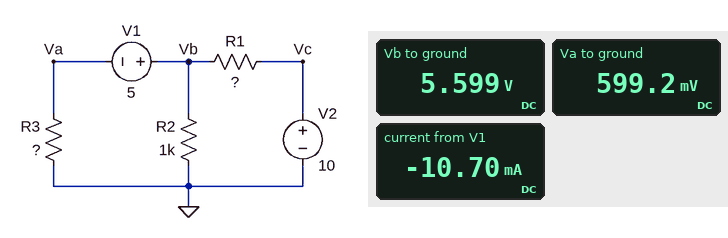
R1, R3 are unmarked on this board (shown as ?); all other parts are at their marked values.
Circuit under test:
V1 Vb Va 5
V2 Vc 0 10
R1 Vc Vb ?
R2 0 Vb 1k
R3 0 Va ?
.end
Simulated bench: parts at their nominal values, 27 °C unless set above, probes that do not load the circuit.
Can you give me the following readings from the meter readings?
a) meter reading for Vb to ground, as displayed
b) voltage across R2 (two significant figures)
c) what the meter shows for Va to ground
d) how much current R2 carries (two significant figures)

5.599 V
5.6 V
599.2 mV
5.6 mA
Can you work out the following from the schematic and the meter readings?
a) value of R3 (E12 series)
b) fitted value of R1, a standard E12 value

56 Ω
270 Ω
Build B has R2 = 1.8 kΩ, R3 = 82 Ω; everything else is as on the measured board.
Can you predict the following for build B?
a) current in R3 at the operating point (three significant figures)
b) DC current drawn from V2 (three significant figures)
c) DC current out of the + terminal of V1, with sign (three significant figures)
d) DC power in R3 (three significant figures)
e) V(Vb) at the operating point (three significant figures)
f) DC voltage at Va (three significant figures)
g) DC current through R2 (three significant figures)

11.7 mA
15.0 mA
-11.7 mA
11.2 mW
5.96 V
957 mV
3.31 mA
